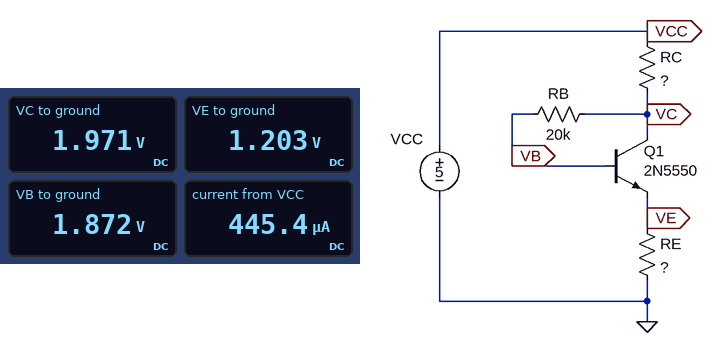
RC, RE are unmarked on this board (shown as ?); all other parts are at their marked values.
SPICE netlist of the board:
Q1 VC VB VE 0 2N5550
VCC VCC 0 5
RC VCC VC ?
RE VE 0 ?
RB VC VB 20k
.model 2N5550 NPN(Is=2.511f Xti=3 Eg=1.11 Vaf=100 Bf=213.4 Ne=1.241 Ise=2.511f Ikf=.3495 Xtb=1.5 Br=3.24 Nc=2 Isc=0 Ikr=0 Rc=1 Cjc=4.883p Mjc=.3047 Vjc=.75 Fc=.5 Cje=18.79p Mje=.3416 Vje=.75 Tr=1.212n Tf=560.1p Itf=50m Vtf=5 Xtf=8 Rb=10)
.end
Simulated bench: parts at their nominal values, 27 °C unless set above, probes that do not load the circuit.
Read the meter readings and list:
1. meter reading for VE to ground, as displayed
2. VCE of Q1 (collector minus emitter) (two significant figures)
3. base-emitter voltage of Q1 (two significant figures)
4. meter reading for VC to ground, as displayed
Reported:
1.203 V
770 mV
670 mV
1.971 V
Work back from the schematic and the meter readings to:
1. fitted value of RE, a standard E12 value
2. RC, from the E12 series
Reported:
2.7 kΩ
6.8 kΩ
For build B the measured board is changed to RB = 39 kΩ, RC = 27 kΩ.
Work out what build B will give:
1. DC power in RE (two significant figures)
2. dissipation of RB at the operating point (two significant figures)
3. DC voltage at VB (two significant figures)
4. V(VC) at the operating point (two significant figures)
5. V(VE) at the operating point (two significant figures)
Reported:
56 µW
130 nW
1.0 V
1.1 V
390 mV
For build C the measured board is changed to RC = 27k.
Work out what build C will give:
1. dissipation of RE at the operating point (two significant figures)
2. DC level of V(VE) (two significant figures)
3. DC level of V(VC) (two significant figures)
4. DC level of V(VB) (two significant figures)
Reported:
57 µW
390 mV
1.1 V
1.0 V
